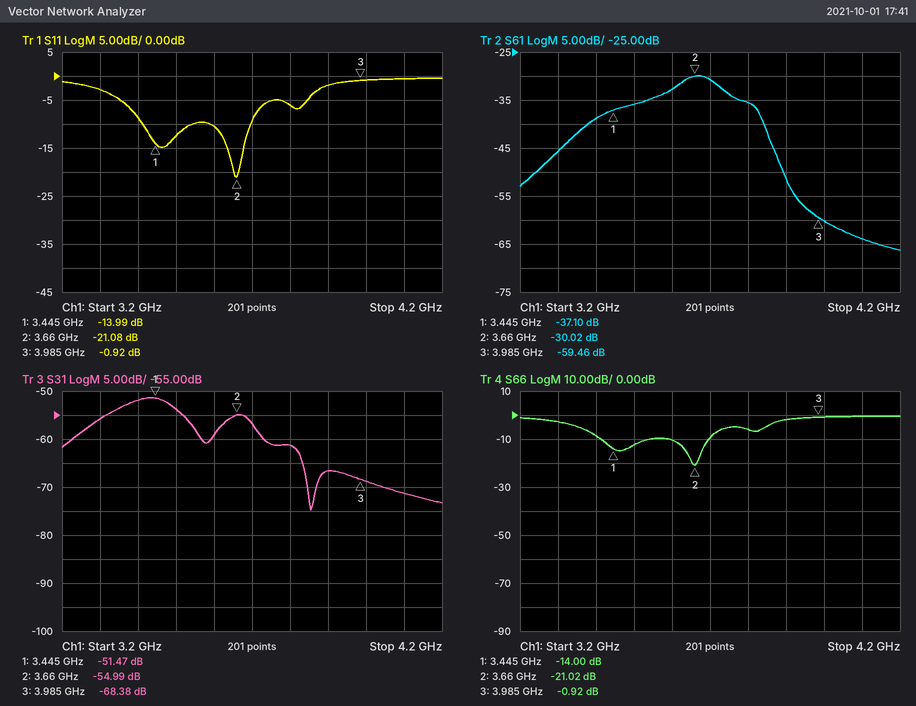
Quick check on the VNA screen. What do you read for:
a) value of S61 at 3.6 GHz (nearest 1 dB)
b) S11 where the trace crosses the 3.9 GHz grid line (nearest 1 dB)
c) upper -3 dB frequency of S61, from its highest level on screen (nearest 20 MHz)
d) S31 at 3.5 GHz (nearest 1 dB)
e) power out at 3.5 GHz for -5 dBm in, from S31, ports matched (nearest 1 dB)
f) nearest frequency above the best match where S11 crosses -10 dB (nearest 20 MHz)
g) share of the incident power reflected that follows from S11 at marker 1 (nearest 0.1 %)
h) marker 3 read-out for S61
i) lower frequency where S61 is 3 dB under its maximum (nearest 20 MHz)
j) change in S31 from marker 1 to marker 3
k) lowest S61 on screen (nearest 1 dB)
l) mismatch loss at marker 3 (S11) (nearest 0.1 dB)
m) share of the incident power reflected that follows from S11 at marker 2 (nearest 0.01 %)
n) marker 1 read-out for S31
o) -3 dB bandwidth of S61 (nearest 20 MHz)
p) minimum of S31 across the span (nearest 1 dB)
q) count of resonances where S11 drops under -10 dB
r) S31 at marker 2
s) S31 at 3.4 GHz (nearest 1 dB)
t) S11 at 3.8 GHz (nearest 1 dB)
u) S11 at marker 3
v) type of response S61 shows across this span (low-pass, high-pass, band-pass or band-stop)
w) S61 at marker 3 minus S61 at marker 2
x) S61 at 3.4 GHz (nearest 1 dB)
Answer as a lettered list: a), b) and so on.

a) -33 dB
b) -2 dB
c) 3.74 GHz
d) -54 dB
e) -59 dBm
f) 3.70 GHz
g) 4.0 %
h) -59.46 dB
i) 3.60 GHz
j) -16.91 dB
k) -66 dB
l) 7.2 dB
m) 0.78 %
n) -51.47 dB
o) 140 MHz
p) -75 dB
q) 2
r) -54.99 dB
s) -52 dB
t) -6 dB
u) -0.92 dB
v) band-pass
w) -29.44 dB
x) -39 dB
